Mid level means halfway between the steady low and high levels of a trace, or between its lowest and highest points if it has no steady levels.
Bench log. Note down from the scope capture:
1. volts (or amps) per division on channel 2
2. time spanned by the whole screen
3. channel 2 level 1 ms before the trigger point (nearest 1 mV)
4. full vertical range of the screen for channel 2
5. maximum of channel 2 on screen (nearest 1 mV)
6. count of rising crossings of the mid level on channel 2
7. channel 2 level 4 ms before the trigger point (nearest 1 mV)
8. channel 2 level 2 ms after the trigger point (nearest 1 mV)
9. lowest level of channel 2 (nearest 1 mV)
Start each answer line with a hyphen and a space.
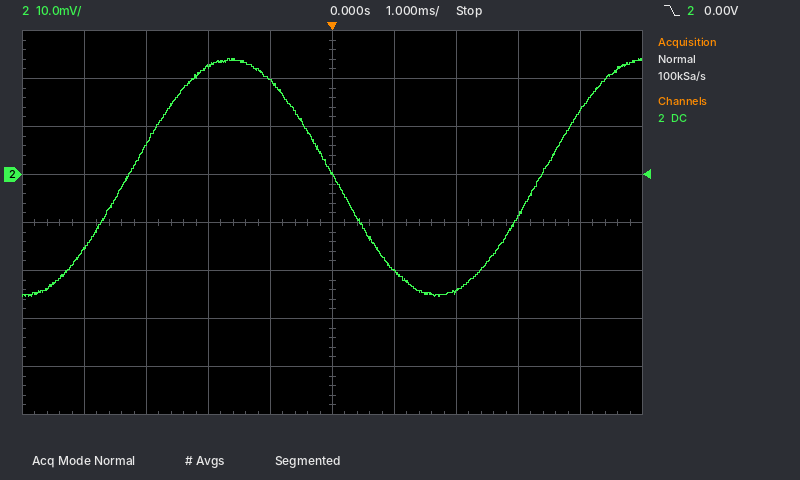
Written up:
- 10 mV
- 10 ms
- 20 mV
- 80 mV
- 24 mV
- 2
- -16 mV
- -24 mV
- -25 mV
